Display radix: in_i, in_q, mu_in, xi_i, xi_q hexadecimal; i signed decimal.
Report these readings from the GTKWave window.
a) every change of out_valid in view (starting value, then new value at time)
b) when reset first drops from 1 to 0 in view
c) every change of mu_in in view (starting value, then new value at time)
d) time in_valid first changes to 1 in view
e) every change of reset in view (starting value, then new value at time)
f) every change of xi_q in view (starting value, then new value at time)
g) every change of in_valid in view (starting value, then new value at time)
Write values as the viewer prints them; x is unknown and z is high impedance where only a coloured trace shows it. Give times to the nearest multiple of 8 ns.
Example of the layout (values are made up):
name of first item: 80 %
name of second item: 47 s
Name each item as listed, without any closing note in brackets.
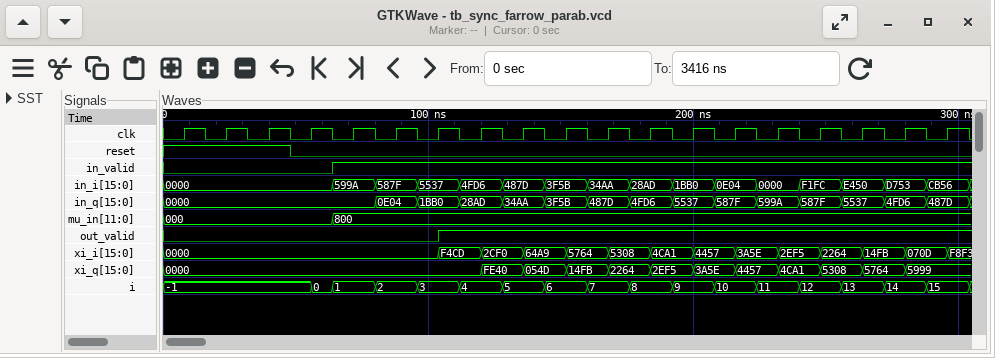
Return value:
every change of out_valid in view: 0, 1 at 104 ns
when reset first drops from 1 to 0 in view: 48 ns
every change of mu_in in view: 000, 800 at 64 ns
time in_valid first changes to 1 in view: 64 ns
every change of reset in view: 1, 0 at 48 ns
every change of xi_q in view: 0000, FE40 at 120 ns, 054D at 136 ns, 14FB at 152 ns, 2264 at 168 ns, 2EF5 at 184 ns, 3A5E at 200 ns, 4457 at 216 ns, 4CA1 at 232 ns, 5308 at 248 ns, 5764 at 264 ns, 5999 at 280 ns
every change of in_valid in view: 0, 1 at 64 ns
